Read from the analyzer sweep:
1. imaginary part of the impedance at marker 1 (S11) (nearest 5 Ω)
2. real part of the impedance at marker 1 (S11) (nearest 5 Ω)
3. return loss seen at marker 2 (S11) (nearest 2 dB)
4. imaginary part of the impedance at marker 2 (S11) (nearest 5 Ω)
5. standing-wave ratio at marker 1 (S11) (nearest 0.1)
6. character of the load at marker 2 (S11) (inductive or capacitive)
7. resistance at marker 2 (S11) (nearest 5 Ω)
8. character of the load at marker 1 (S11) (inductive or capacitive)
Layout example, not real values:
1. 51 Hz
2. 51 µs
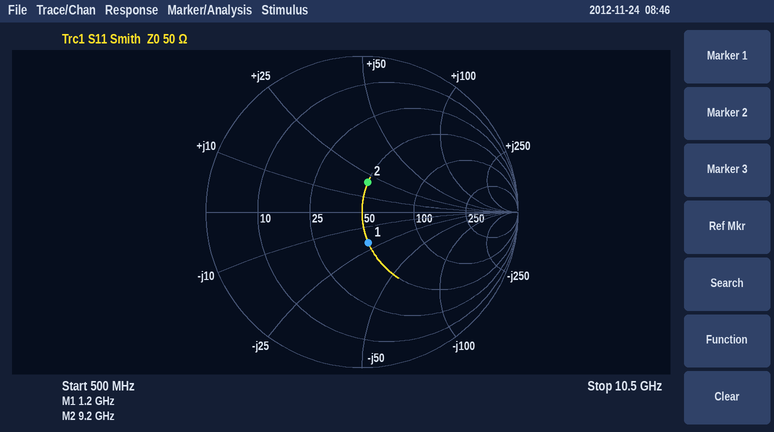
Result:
1. -20 Ω
2. 50 Ω
3. 14 dB
4. +20 Ω
5. 1.5
6. inductive
7. 50 Ω
8. capacitive
